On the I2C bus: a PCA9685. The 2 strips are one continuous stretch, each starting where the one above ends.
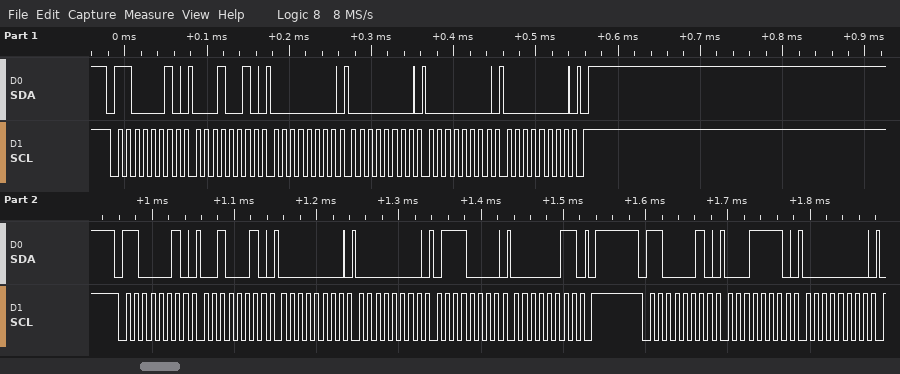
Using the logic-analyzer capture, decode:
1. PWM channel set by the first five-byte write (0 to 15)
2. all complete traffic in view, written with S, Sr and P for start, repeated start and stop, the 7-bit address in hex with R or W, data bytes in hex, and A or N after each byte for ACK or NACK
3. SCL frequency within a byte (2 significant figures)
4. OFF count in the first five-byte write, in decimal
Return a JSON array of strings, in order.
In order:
["3", "S 61W A 12 A 00 A 00 A 00 A 00 A P S 61W A 22 A 00 A 00 A 70 A 03 A P S 61W A 1E A 00 A", "100 kHz", "0"]
